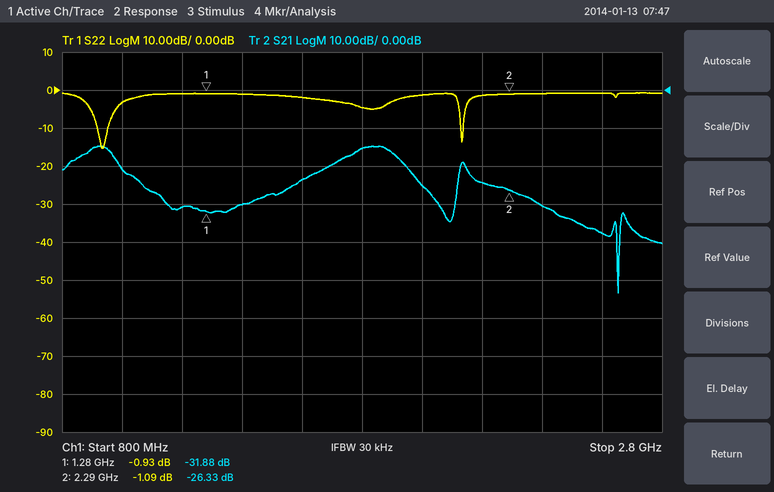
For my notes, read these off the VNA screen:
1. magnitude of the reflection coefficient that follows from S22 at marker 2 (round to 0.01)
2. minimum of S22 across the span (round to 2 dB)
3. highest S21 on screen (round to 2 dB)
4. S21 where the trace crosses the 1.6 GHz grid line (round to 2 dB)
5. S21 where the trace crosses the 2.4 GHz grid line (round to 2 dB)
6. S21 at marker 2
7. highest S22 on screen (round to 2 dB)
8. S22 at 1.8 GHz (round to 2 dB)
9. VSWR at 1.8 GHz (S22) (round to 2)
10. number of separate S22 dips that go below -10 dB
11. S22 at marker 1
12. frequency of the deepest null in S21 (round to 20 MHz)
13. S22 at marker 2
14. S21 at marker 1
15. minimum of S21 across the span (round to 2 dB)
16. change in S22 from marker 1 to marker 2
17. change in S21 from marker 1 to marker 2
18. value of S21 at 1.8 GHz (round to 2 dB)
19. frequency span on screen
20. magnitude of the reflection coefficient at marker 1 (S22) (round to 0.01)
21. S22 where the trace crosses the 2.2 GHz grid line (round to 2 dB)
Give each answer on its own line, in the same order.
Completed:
0.88
-16 dB
-14 dB
-24 dB
-30 dB
-26.33 dB
0 dB
-4 dB
4
2
-0.93 dB
2.66 GHz
-1.09 dB
-31.88 dB
-54 dB
-0.16 dB
5.55 dB
-16 dB
2 GHz
0.90
-2 dB
